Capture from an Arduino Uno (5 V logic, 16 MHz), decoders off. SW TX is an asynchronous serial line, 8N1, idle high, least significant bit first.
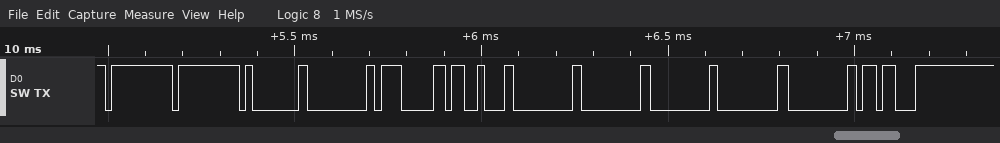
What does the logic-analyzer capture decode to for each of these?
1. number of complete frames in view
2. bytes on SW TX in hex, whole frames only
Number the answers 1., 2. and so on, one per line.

1. 12
2. 0xFF 0xFF 0x01 0x00 0x07 0x13 0x00 0x00 0x00 0x00 0x00 0x1B
